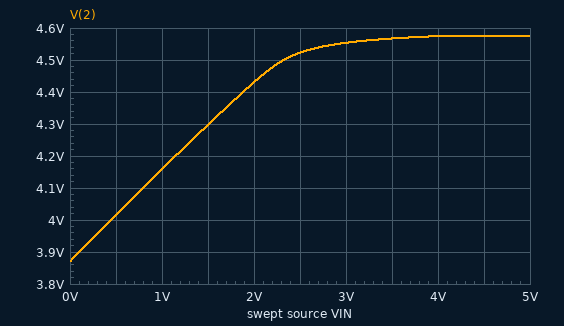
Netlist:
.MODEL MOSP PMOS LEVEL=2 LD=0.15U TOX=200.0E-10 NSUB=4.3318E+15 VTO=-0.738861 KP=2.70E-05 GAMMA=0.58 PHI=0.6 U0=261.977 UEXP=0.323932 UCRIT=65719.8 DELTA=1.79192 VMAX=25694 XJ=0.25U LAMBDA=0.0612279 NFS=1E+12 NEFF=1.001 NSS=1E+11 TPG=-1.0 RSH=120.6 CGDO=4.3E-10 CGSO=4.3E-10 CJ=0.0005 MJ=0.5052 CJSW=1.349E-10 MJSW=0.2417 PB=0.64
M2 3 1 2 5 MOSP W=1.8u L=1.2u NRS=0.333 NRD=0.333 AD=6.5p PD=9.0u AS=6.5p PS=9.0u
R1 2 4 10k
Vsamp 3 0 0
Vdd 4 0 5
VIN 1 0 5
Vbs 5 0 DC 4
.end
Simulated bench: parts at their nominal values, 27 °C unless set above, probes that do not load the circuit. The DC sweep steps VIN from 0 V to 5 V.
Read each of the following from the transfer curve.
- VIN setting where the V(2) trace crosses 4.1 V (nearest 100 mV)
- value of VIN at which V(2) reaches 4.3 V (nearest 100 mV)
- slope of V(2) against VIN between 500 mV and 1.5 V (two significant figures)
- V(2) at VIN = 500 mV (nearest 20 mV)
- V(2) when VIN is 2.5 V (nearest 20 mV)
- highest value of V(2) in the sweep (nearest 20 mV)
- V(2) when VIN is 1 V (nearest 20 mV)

800 mV
1.5 V
0.28 V/V
4.02 V
4.52 V
4.58 V
4.16 V
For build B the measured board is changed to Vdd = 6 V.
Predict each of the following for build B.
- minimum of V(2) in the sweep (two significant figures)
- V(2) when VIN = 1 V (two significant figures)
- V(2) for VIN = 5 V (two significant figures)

4.5 V
4.6 V
4.6 V
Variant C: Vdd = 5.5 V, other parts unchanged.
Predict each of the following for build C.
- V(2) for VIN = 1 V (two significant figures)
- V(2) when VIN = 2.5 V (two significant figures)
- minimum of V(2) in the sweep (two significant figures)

4.5 V
4.6 V
4.2 V
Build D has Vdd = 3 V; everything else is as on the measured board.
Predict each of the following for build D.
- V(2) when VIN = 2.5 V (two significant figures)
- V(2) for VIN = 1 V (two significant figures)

3.0 V
2.8 V
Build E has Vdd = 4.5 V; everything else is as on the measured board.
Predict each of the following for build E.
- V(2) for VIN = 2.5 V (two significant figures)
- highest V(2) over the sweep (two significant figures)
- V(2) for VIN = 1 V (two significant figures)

4.2 V
4.5 V
3.8 V
